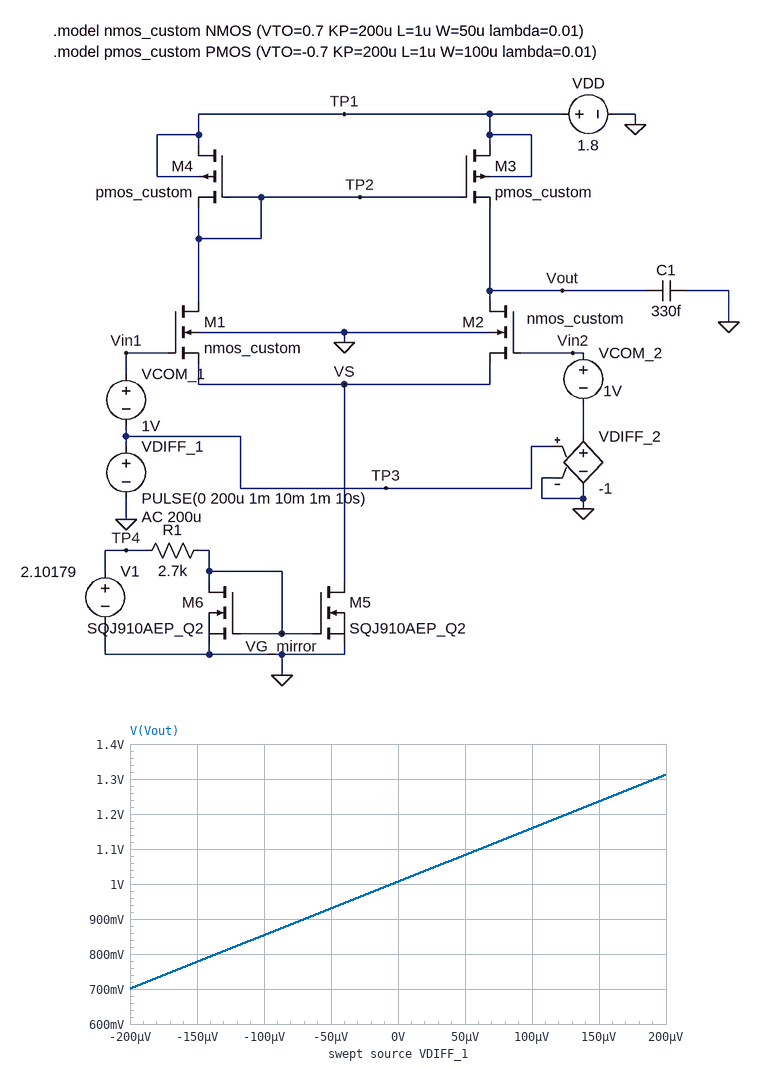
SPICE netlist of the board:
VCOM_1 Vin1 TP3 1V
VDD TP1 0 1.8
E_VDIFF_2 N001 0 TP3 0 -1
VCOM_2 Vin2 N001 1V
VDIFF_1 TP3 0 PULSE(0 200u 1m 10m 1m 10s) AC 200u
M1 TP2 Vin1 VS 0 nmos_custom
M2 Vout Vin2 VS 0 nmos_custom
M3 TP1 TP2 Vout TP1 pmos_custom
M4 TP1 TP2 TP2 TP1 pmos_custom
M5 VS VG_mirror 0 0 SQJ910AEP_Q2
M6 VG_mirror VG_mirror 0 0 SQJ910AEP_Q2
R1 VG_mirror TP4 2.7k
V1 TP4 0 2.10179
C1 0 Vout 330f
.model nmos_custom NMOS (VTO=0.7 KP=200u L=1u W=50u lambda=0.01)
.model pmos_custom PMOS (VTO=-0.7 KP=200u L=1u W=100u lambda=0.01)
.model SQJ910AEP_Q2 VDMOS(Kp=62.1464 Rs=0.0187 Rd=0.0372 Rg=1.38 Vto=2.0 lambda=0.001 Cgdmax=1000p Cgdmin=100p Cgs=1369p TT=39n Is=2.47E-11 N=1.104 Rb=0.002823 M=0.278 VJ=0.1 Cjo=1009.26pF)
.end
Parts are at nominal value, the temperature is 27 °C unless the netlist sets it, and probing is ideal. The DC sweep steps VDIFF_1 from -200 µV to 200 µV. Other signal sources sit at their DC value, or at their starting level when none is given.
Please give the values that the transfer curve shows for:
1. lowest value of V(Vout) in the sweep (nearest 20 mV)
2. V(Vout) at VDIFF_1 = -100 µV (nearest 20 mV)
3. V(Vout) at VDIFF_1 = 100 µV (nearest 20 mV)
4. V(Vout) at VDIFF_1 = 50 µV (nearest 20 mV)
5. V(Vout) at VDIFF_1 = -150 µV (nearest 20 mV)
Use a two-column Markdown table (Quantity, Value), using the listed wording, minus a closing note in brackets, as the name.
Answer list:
| Quantity | Value |
|---|---|
| lowest value of V(Vout) in the sweep | 700 mV |
| V(Vout) at VDIFF_1 = -100 µV | 860 mV |
| V(Vout) at VDIFF_1 = 100 µV | 1.16 V |
| V(Vout) at VDIFF_1 = 50 µV | 1.08 V |
| V(Vout) at VDIFF_1 = -150 µV | 780 mV |
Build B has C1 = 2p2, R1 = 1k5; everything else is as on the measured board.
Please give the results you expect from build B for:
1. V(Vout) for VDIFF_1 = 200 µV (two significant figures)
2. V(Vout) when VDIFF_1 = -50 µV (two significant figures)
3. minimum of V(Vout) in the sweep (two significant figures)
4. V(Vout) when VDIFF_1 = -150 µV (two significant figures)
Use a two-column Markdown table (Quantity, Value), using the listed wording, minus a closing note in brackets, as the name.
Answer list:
| Quantity | Value |
|---|---|
| V(Vout) for VDIFF_1 = 200 µV | 1.2 V |
| V(Vout) when VDIFF_1 = -50 µV | 920 mV |
| minimum of V(Vout) in the sweep | 740 mV |
| V(Vout) when VDIFF_1 = -150 µV | 800 mV |
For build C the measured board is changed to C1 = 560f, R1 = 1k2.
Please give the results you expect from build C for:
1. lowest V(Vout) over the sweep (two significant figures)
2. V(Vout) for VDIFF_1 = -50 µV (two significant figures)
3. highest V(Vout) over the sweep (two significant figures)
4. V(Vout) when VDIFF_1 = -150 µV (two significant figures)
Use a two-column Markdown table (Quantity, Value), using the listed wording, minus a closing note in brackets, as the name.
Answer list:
| Quantity | Value |
|---|---|
| lowest V(Vout) over the sweep | 750 mV |
| V(Vout) for VDIFF_1 = -50 µV | 910 mV |
| highest V(Vout) over the sweep | 1.2 V |
| V(Vout) when VDIFF_1 = -150 µV | 810 mV |
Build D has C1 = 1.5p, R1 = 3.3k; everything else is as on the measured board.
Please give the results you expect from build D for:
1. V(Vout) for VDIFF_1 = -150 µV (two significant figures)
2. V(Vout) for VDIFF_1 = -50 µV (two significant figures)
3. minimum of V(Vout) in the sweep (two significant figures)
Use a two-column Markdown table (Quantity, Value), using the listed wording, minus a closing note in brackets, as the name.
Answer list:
| Quantity | Value |
|---|---|
| V(Vout) for VDIFF_1 = -150 µV | 760 mV |
| V(Vout) for VDIFF_1 = -50 µV | 930 mV |
| minimum of V(Vout) in the sweep | 680 mV |
